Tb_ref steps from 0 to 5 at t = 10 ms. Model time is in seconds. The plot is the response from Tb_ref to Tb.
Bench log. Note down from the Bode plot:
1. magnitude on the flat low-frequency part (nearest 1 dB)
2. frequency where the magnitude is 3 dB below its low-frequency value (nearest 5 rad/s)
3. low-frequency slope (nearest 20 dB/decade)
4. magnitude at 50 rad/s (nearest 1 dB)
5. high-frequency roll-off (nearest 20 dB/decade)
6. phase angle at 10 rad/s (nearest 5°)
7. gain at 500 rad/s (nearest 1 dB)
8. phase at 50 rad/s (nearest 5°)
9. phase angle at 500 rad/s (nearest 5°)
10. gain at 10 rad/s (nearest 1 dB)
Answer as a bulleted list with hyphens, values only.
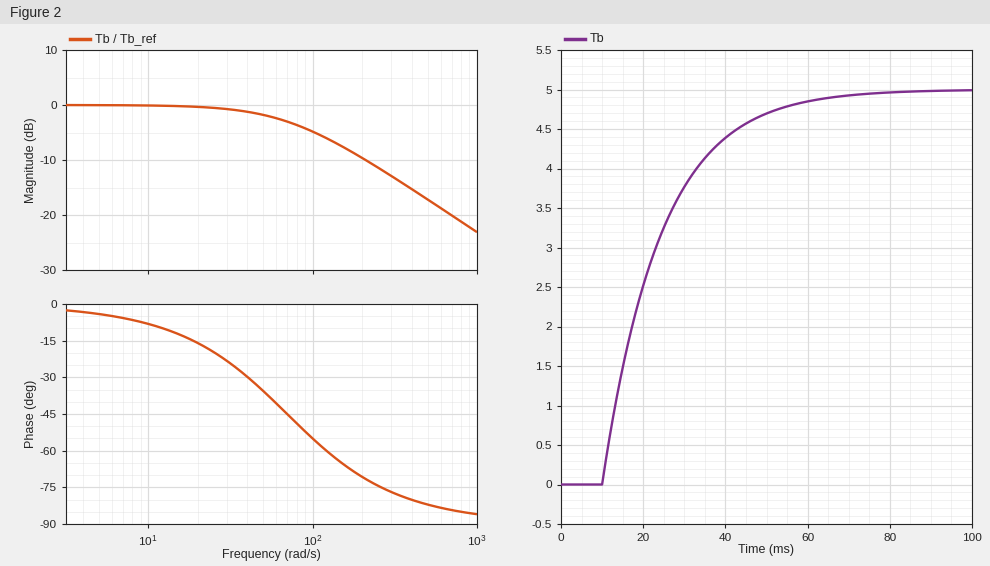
- 0 dB
- 70 rad/s
- 0 dB/decade
- -2 dB
- -20 dB/decade
- -10°
- -17 dB
- -35°
- -80°
- 0 dB
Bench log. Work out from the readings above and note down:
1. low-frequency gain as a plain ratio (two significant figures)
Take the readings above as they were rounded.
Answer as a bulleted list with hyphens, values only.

- 1.0
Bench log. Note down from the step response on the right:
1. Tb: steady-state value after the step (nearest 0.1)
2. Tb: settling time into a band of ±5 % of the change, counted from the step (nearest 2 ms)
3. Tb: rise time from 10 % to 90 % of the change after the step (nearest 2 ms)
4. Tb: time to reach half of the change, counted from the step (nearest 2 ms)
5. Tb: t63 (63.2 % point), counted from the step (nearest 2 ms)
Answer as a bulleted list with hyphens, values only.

- 5.0
- 42 ms
- 32 ms
- 10 ms
- 14 ms
